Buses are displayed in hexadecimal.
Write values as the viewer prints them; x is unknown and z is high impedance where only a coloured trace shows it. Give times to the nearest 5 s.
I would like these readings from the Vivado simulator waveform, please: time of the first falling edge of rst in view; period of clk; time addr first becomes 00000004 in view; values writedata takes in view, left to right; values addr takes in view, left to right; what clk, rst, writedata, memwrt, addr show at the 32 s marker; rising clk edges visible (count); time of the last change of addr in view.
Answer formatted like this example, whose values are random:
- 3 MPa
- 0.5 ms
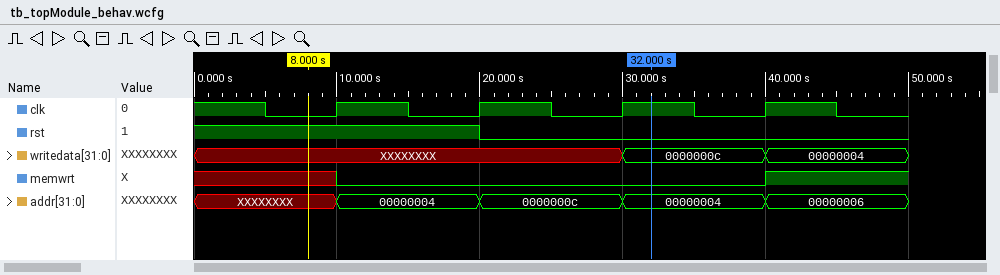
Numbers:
- 20 s
- 10 s
- 10 s
- XXXXXXXX, 0000000c, 00000004
- XXXXXXXX, 00000004, 0000000c, 00000004, 00000006
- clk=1, rst=0, writedata=0000000c, memwrt=0, addr=00000004
- 4
- 40 s
